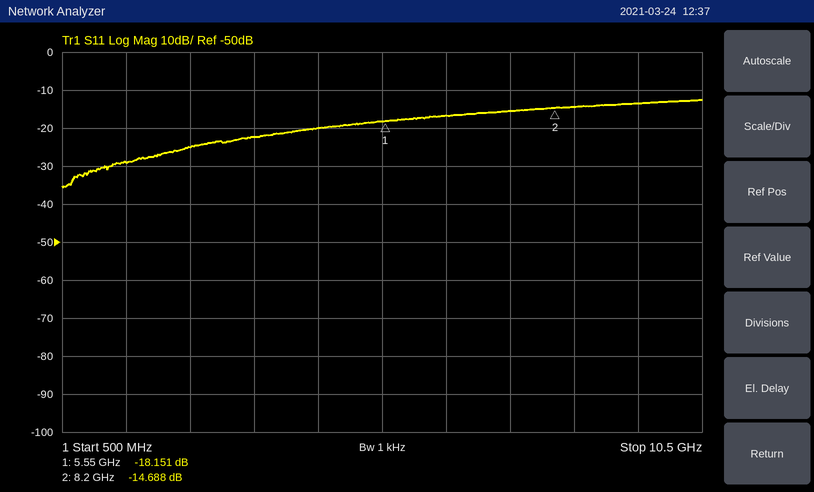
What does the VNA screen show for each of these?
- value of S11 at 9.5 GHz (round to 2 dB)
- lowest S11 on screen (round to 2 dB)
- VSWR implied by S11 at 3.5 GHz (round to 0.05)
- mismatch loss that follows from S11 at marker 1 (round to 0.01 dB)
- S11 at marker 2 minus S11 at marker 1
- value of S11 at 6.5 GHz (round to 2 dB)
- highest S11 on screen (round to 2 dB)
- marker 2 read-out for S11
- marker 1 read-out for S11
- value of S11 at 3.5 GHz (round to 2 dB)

-14 dB
-36 dB
1.15
0.07 dB
3.463 dB
-16 dB
-12 dB
-14.688 dB
-18.151 dB
-22 dB
